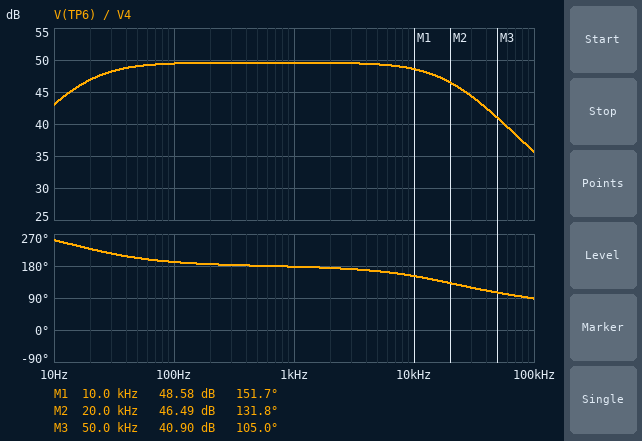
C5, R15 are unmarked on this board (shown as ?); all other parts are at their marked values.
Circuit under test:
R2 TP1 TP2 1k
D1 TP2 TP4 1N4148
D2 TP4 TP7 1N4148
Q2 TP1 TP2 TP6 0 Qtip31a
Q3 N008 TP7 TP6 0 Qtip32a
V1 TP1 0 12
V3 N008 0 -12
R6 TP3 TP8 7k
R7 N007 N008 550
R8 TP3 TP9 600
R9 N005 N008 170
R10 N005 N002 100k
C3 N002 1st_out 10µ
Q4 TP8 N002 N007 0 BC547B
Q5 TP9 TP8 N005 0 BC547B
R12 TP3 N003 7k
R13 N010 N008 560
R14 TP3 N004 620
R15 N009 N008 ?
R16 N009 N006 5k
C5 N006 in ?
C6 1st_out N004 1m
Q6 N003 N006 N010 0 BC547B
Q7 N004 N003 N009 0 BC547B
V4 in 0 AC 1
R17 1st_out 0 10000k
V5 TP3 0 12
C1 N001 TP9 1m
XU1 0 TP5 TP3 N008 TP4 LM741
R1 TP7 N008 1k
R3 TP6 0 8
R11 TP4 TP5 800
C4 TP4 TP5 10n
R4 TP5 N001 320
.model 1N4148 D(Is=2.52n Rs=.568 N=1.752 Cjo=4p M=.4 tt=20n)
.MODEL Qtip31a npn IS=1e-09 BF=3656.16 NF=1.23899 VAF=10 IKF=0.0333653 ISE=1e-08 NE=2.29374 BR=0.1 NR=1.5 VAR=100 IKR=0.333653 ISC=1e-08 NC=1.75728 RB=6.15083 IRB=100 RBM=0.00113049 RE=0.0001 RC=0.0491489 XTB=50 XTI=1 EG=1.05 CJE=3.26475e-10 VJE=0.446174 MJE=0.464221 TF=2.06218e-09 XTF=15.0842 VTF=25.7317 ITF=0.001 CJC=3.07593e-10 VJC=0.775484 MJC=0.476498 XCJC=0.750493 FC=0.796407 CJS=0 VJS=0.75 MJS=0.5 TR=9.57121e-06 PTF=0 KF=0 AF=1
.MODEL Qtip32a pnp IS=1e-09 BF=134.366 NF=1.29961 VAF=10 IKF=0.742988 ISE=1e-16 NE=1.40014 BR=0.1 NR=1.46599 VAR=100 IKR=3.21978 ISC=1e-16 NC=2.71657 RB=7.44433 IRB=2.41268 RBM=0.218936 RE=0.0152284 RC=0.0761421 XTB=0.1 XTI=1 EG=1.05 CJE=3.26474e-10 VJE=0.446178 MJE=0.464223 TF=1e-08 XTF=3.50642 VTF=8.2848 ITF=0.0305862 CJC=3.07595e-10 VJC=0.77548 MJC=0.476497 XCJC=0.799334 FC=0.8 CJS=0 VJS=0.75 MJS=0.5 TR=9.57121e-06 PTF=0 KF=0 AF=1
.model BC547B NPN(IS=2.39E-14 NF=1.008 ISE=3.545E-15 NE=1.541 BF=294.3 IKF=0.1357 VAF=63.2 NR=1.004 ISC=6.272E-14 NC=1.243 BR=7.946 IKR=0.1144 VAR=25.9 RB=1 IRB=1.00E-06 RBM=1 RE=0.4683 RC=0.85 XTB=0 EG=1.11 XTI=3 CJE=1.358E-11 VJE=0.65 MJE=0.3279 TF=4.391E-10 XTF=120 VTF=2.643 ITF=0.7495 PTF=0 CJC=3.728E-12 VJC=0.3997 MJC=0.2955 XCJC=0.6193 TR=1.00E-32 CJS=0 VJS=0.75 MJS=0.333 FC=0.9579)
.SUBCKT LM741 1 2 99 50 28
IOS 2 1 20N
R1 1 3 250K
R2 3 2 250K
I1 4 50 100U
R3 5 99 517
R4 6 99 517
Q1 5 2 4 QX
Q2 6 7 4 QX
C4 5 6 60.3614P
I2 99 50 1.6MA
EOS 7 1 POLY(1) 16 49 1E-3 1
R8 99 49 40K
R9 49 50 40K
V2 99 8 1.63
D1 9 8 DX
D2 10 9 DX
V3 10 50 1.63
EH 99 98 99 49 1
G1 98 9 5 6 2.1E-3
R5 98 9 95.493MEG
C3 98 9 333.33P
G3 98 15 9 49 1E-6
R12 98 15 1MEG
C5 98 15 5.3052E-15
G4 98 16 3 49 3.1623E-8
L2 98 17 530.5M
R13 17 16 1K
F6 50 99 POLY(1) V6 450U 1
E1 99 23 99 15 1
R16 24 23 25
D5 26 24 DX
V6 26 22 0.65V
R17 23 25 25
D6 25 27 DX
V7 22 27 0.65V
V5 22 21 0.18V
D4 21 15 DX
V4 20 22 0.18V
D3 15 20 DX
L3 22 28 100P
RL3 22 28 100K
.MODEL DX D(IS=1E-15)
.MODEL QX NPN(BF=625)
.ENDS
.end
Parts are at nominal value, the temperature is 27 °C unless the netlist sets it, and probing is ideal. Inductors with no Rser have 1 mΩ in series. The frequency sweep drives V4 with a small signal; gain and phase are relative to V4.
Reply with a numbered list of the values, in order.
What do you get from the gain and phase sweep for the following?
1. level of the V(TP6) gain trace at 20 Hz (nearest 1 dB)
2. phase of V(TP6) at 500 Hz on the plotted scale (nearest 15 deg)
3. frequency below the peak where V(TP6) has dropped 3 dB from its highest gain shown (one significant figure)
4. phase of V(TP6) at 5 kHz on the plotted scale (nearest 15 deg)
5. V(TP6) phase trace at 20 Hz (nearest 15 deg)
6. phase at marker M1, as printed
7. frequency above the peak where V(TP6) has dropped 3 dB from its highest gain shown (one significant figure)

1. 47 dB
2. 180 deg
3. 20 Hz
4. 165 deg
5. 225 deg
6. 151.7 deg
7. 20 kHz
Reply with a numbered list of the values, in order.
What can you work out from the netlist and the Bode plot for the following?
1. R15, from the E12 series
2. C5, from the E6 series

1. 820 Ω
2. 22 µF
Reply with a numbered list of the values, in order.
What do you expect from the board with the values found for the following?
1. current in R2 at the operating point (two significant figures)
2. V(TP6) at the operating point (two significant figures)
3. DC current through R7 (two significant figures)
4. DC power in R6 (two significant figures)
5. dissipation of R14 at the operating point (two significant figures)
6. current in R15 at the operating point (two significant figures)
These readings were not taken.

1. 11 mA
2. -2.9 mV
3. 2.8 mA
4. 58 mW
5. 5.3 mW
6. 2.9 mA
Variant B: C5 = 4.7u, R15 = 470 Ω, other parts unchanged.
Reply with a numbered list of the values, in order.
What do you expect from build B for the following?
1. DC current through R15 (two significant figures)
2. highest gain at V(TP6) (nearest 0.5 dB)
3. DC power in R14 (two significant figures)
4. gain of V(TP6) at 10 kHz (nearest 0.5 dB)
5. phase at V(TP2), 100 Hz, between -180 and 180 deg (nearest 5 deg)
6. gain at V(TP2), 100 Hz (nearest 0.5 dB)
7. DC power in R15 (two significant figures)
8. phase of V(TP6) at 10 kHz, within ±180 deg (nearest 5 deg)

1. 5.1 mA
2. 53.5 dB
3. 16 mW
4. 52.5 dB
5. -140 deg
6. 51.5 dB
7. 12 mW
8. 150 deg
